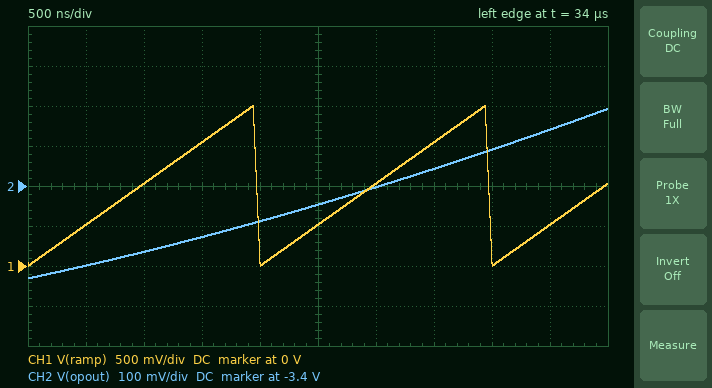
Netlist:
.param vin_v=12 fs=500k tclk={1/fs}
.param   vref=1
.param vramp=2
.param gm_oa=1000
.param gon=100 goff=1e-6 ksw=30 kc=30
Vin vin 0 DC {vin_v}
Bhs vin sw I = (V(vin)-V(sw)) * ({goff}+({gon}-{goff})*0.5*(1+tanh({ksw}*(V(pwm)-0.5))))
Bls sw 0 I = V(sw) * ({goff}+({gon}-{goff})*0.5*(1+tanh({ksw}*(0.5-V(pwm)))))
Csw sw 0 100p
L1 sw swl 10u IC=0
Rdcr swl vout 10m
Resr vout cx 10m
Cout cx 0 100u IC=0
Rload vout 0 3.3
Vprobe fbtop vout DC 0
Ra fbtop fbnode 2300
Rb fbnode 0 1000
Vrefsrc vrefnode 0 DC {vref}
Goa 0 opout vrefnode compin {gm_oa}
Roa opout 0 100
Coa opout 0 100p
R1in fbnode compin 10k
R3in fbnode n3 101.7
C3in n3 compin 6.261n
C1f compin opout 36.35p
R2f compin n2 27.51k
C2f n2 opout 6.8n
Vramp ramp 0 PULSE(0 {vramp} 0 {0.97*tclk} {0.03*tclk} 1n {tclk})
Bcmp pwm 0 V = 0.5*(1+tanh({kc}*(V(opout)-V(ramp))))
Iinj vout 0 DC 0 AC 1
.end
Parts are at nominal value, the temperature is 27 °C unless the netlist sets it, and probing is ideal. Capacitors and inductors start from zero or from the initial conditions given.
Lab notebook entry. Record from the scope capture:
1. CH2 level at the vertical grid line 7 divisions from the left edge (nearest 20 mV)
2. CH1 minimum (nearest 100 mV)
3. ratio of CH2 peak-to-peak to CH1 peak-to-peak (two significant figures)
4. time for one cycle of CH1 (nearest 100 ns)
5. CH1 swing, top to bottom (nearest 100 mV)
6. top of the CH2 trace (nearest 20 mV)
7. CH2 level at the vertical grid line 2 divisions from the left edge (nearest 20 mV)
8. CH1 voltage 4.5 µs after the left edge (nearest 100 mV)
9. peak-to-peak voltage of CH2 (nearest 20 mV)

-3.36 V
0 V
0.21
2.0 µs
2.0 V
-3.20 V
-3.56 V
500 mV
420 mV
